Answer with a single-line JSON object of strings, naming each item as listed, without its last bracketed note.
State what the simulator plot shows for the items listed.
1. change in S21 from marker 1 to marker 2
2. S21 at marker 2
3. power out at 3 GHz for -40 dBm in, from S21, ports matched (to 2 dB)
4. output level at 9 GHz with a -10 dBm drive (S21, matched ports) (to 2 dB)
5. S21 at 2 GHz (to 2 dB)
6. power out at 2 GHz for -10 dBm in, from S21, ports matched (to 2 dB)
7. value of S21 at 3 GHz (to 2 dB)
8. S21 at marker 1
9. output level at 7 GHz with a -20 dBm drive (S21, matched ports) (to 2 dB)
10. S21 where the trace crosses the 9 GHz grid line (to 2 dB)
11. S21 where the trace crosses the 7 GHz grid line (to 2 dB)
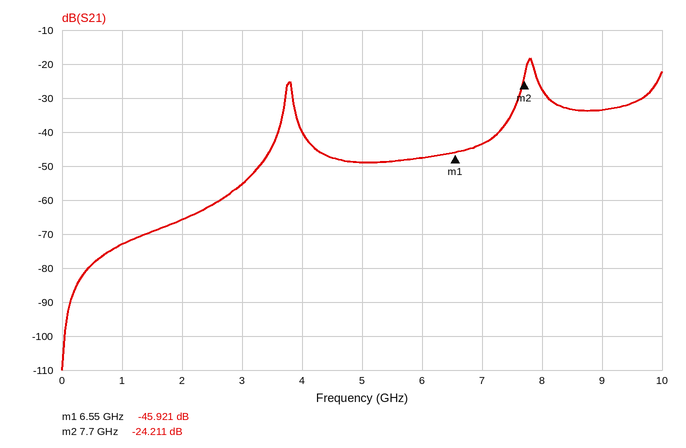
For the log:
{"change in S21 from marker 1 to marker 2": "21.710 dB", "S21 at marker 2": "-24.211 dB", "power out at 3 GHz for -40 dBm in, from S21, ports matched": "-96 dBm", "output level at 9 GHz with a -10 dBm drive (S21, matched ports)": "-44 dBm", "S21 at 2 GHz": "-66 dB", "power out at 2 GHz for -10 dBm in, from S21, ports matched": "-76 dBm", "value of S21 at 3 GHz": "-56 dB", "S21 at marker 1": "-45.921 dB", "output level at 7 GHz with a -20 dBm drive (S21, matched ports)": "-64 dBm", "S21 where the trace crosses the 9 GHz grid line": "-34 dB", "S21 where the trace crosses the 7 GHz grid line": "-44 dB"}
